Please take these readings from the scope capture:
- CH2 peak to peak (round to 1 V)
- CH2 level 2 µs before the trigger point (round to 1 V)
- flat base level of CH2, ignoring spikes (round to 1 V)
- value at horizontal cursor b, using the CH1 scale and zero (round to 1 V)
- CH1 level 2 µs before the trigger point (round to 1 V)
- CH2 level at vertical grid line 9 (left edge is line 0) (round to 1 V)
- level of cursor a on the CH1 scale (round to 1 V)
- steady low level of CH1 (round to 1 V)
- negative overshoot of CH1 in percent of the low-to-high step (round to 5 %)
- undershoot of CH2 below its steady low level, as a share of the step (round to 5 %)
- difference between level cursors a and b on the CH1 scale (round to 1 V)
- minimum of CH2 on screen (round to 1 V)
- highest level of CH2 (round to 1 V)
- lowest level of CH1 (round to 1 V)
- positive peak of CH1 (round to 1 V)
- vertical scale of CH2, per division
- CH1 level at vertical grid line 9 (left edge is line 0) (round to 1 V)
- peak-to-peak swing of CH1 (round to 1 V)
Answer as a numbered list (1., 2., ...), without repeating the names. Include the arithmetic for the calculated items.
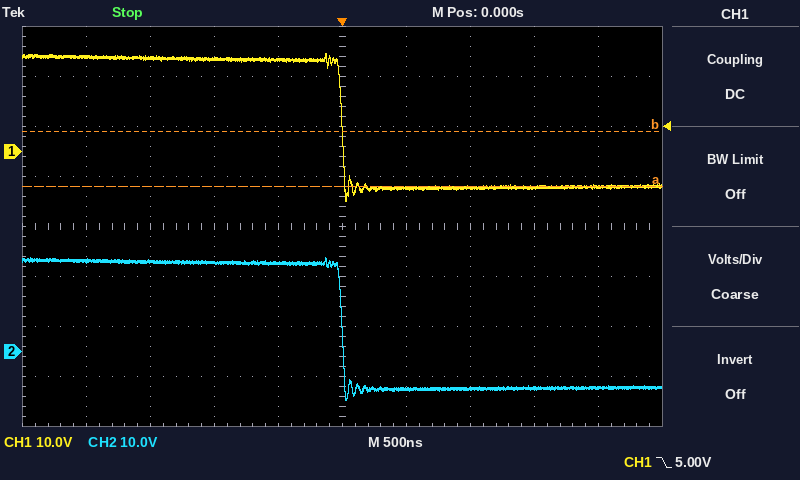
1. 19 V − (-10 V) = 29 V
2. 18 V
3. -7 V
4. 4 V
5. 19 V
6. -7 V
7. -7 V
8. -7 V
9. 10 %
10. 10 %
11. 11 V
12. -10 V
13. 19 V
14. -10 V
15. 20 V
16. 10 V
17. -7 V
18. 20 V − (-10 V) = 30 V
